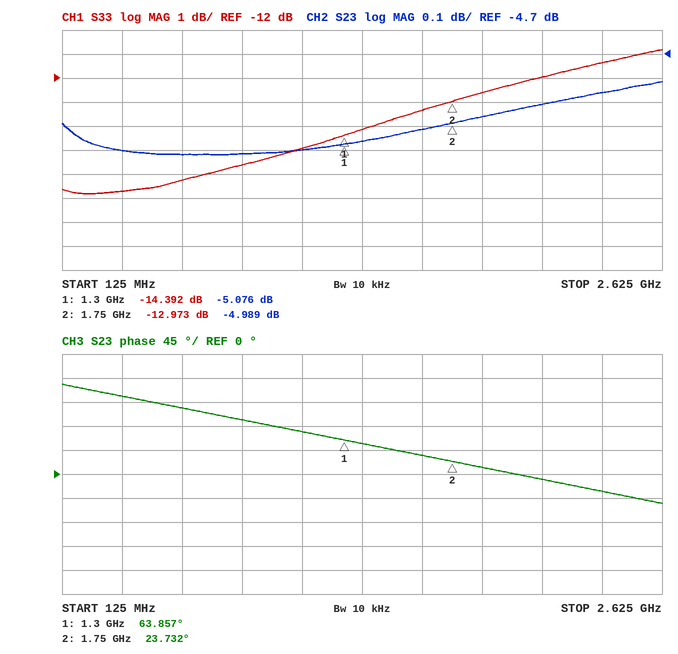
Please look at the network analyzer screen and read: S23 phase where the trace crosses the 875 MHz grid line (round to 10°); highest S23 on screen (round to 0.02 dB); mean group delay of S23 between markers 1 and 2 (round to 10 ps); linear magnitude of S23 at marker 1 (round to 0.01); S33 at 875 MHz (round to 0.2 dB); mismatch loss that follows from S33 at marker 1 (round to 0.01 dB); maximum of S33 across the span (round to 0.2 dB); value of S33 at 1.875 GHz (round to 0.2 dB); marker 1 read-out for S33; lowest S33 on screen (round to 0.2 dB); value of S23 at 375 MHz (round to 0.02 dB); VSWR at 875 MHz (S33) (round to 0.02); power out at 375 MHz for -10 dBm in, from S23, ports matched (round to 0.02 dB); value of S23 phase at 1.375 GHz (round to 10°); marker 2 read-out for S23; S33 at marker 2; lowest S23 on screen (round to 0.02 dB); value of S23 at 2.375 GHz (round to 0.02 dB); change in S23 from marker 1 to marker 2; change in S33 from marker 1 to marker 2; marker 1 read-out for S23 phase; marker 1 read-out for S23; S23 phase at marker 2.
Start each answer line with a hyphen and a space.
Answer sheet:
- 100°
- -4.82 dB
- 250 ps
- 0.56
- -15.6 dB
- 0.16 dB
- -10.8 dB
- -12.6 dB
- -14.392 dB
- -16.8 dB
- -5.10 dB
- 1.40
- -15.10 dBm
- 60°
- -4.989 dB
- -12.973 dB
- -5.12 dB
- -4.86 dB
- 0.087 dB
- 1.419 dB
- 63.857°
- -5.076 dB
- 23.732°
